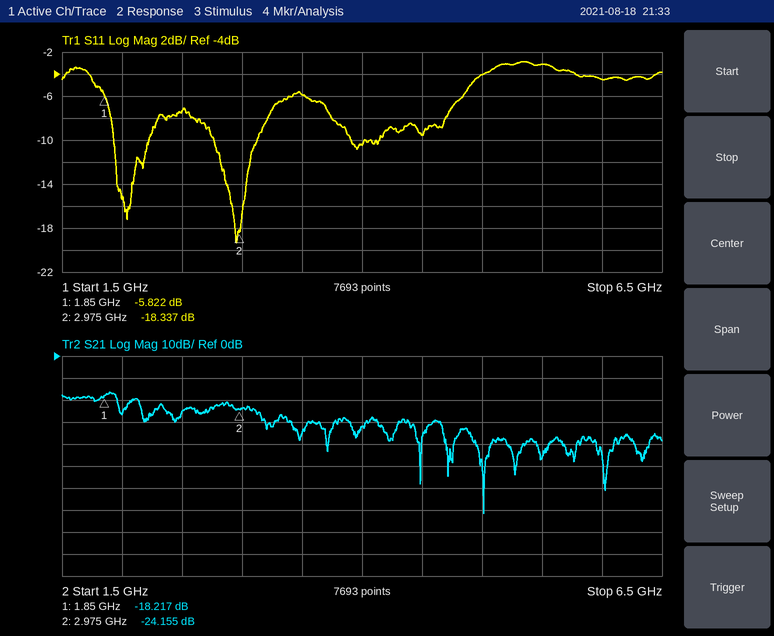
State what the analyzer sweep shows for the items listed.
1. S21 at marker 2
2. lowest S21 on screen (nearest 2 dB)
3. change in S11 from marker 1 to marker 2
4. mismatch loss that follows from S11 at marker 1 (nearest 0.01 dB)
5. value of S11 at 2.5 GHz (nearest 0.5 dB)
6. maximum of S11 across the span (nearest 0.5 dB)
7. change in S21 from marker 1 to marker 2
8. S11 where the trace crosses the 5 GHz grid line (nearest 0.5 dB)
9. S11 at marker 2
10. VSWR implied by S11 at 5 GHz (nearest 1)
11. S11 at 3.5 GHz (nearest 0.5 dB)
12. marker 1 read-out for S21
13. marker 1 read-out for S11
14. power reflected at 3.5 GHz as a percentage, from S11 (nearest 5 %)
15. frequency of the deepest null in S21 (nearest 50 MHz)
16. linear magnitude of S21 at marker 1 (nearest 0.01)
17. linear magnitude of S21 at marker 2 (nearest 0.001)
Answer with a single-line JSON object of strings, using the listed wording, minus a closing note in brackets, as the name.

{"S21 at marker 2": "-24.155 dB", "lowest S21 on screen": "-72 dB", "change in S11 from marker 1 to marker 2": "-12.515 dB", "mismatch loss that follows from S11 at marker 1": "1.32 dB", "value of S11 at 2.5 GHz": "-7.5 dB", "maximum of S11 across the span": "-3.0 dB", "change in S21 from marker 1 to marker 2": "-5.938 dB", "S11 where the trace crosses the 5 GHz grid line": "-4.0 dB", "S11 at marker 2": "-18.337 dB", "VSWR implied by S11 at 5 GHz": "4", "S11 at 3.5 GHz": "-6.0 dB", "marker 1 read-out for S21": "-18.217 dB", "marker 1 read-out for S11": "-5.822 dB", "power reflected at 3.5 GHz as a percentage, from S11": "25 %", "frequency of the deepest null in S21": "5.00 GHz", "linear magnitude of S21 at marker 1": "0.12", "linear magnitude of S21 at marker 2": "0.062"}
